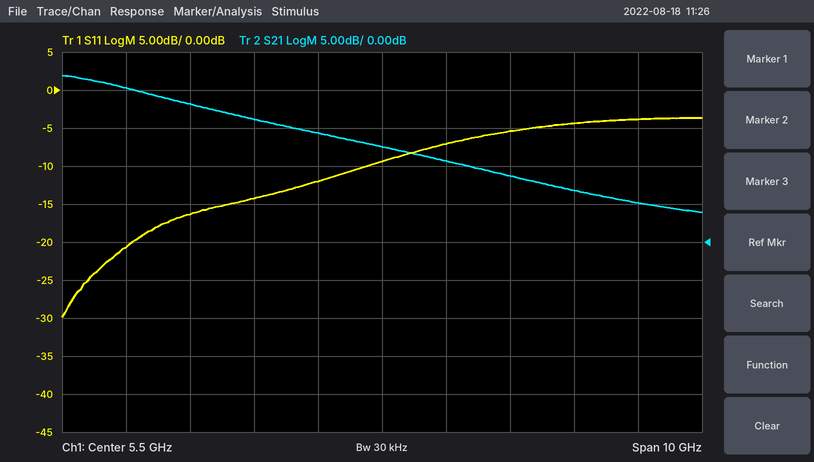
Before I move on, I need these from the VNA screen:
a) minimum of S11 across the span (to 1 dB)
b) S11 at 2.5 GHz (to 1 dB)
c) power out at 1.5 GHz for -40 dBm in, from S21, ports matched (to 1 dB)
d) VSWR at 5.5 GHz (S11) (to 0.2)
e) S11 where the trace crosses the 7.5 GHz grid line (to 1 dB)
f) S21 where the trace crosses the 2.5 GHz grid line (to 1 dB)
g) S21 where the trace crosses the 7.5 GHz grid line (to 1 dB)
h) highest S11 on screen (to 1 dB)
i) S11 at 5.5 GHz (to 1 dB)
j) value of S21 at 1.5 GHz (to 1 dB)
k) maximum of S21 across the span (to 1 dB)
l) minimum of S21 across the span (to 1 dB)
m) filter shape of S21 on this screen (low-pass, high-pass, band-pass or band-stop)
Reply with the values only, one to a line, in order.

-30 dB
-16 dB
-20 dBm
2.0
-5 dB
18 dB
9 dB
-4 dB
-9 dB
20 dB
22 dB
4 dB
low-pass
